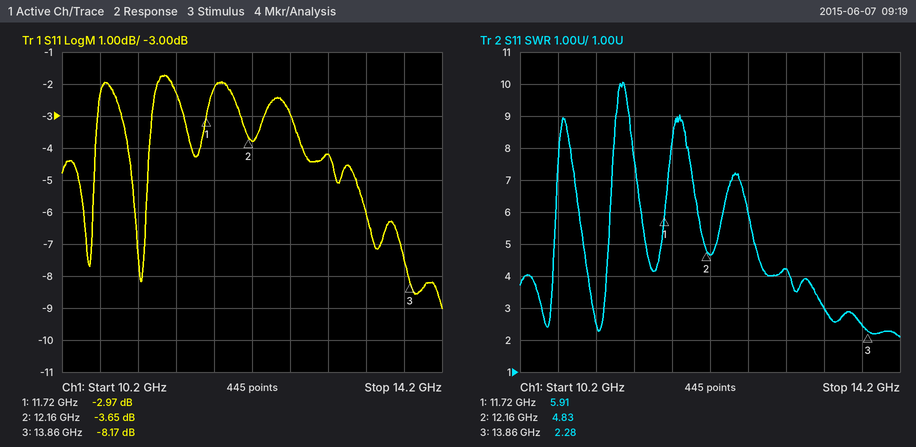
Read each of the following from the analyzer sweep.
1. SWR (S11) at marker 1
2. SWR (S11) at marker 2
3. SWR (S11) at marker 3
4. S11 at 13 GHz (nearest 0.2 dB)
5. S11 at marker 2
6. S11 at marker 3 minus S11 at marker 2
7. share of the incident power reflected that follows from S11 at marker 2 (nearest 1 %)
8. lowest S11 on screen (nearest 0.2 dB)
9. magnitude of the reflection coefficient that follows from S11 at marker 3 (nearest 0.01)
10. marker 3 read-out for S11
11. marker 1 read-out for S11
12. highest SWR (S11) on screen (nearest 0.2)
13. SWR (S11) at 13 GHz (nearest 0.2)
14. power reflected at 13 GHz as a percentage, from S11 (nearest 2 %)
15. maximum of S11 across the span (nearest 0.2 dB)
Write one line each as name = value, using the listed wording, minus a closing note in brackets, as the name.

SWR (S11) at marker 1 = 5.91
SWR (S11) at marker 2 = 4.83
SWR (S11) at marker 3 = 2.28
S11 at 13 GHz = -4.2 dB
S11 at marker 2 = -3.65 dB
S11 at marker 3 minus S11 at marker 2 = -4.52 dB
share of the incident power reflected that follows from S11 at marker 2 = 43 %
lowest S11 on screen = -9.0 dB
magnitude of the reflection coefficient that follows from S11 at marker 3 = 0.39
marker 3 read-out for S11 = -8.17 dB
marker 1 read-out for S11 = -2.97 dB
highest SWR (S11) on screen = 10.0
SWR (S11) at 13 GHz = 4.2
power reflected at 13 GHz as a percentage, from S11 = 38 %
maximum of S11 across the span = -1.8 dB
